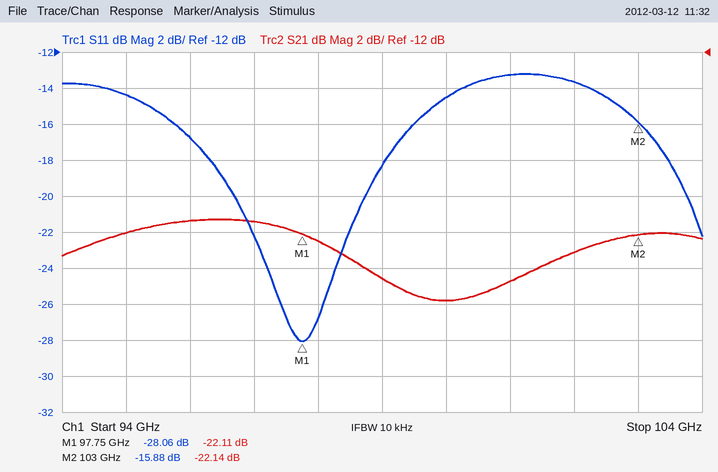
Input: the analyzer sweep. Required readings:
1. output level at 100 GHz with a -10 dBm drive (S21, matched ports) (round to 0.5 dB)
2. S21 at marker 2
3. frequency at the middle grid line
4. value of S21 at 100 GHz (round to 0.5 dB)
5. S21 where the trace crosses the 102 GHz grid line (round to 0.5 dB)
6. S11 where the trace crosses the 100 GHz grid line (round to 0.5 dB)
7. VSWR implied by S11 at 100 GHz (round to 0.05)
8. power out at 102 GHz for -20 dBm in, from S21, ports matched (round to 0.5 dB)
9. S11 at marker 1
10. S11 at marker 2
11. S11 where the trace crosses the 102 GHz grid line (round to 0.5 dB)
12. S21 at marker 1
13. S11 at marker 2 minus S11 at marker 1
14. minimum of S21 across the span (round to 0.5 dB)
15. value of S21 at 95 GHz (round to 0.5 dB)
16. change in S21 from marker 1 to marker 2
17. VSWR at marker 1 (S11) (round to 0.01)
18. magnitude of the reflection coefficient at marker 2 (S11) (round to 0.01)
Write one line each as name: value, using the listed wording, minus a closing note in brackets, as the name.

output level at 100 GHz with a -10 dBm drive (S21, matched ports): -36.0 dBm
S21 at marker 2: -22.14 dB
frequency at the middle grid line: 99 GHz
value of S21 at 100 GHz: -26.0 dB
S21 where the trace crosses the 102 GHz grid line: -23.0 dB
S11 where the trace crosses the 100 GHz grid line: -14.5 dB
VSWR implied by S11 at 100 GHz: 1.45
power out at 102 GHz for -20 dBm in, from S21, ports matched: -43.0 dBm
S11 at marker 1: -28.06 dB
S11 at marker 2: -15.88 dB
S11 where the trace crosses the 102 GHz grid line: -13.5 dB
S21 at marker 1: -22.11 dB
S11 at marker 2 minus S11 at marker 1: 12.18 dB
minimum of S21 across the span: -26.0 dB
value of S21 at 95 GHz: -22.0 dB
change in S21 from marker 1 to marker 2: -0.03 dB
VSWR at marker 1 (S11): 1.08
magnitude of the reflection coefficient at marker 2 (S11): 0.16
